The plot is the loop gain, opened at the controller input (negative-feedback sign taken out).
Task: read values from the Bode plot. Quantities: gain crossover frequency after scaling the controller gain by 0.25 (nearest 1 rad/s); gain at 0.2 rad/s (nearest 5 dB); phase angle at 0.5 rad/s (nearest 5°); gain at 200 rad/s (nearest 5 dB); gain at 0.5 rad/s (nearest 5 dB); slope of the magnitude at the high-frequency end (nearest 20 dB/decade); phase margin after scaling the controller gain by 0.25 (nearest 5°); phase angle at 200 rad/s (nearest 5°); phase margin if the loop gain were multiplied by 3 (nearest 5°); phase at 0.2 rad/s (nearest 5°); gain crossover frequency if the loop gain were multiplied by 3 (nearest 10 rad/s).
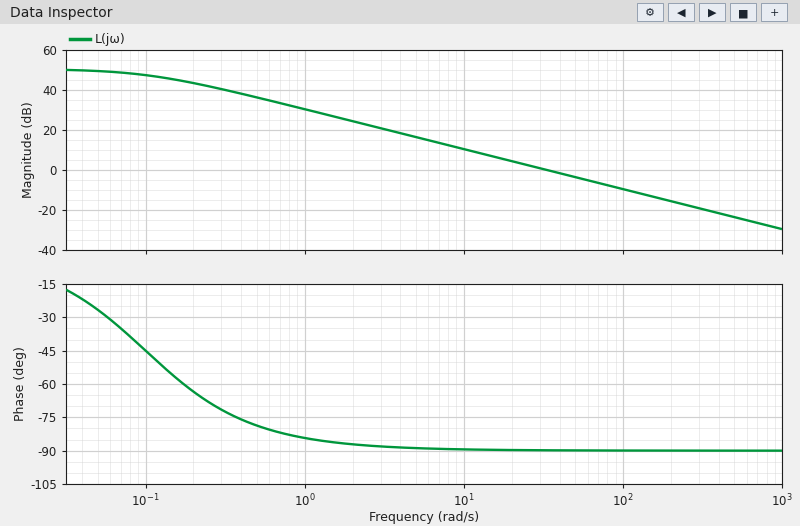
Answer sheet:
8 rad/s
45 dB
-80°
-15 dB
35 dB
-20 dB/decade
90°
-90°
90°
-65°
100 rad/s
